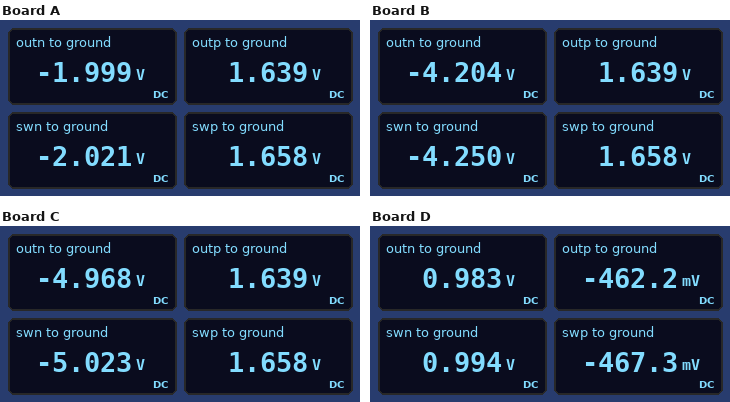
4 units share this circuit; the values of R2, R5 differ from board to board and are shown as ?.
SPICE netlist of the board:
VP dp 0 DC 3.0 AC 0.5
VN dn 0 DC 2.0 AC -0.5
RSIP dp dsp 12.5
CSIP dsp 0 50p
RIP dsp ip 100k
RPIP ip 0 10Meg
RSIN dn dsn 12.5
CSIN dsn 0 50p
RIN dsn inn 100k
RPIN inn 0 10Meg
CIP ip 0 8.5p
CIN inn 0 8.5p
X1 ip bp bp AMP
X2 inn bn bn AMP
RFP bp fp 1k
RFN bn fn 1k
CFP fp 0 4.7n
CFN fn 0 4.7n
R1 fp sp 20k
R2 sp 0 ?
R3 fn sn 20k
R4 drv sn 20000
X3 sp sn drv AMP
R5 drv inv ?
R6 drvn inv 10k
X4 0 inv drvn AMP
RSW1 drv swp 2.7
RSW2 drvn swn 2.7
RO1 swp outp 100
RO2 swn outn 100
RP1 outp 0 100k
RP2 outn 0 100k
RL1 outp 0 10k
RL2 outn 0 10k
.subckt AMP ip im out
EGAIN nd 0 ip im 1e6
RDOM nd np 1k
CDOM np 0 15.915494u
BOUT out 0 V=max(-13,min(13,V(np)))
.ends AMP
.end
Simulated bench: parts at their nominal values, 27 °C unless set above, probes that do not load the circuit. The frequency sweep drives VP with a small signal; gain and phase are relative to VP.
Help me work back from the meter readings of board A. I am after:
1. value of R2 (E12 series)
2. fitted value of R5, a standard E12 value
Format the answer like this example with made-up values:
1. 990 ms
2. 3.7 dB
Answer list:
1. 33 kΩ
2. 8.2 kΩ
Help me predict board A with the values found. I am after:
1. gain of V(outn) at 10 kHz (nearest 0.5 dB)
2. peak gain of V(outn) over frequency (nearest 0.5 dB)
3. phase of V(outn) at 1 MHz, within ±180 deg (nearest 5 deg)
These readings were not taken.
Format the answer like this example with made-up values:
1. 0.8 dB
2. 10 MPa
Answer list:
1. 5.5 dB
2. 6.0 dB
3. -15 deg
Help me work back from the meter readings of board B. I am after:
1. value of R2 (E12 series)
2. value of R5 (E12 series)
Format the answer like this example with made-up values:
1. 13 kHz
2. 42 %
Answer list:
1. 33 kΩ
2. 3.9 kΩ
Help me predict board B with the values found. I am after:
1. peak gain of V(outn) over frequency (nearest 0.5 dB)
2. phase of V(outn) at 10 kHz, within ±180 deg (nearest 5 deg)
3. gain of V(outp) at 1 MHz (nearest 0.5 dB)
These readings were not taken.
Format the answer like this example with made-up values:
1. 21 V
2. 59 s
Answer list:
1. 12.5 dB
2. 160 deg
3. -39.5 dB
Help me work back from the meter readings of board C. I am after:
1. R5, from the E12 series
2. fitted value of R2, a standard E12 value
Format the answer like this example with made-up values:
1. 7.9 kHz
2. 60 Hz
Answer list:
1. 3.3 kΩ
2. 33 kΩ
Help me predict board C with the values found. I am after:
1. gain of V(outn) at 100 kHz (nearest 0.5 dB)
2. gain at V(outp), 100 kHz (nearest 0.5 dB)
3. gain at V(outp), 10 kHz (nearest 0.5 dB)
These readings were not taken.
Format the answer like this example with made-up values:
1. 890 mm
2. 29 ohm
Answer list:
1. 3.5 dB
2. -6.5 dB
3. 4.0 dB
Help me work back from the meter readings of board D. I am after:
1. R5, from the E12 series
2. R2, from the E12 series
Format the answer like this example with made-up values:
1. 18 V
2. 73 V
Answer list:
1. 4.7 kΩ
2. 6.8 kΩ
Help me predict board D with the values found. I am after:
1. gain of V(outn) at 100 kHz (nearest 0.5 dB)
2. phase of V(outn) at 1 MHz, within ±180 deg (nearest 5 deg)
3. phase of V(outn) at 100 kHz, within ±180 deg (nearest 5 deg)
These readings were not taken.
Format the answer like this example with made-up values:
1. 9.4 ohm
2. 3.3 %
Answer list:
1. -4.5 dB
2. -20 deg
3. 80 deg
